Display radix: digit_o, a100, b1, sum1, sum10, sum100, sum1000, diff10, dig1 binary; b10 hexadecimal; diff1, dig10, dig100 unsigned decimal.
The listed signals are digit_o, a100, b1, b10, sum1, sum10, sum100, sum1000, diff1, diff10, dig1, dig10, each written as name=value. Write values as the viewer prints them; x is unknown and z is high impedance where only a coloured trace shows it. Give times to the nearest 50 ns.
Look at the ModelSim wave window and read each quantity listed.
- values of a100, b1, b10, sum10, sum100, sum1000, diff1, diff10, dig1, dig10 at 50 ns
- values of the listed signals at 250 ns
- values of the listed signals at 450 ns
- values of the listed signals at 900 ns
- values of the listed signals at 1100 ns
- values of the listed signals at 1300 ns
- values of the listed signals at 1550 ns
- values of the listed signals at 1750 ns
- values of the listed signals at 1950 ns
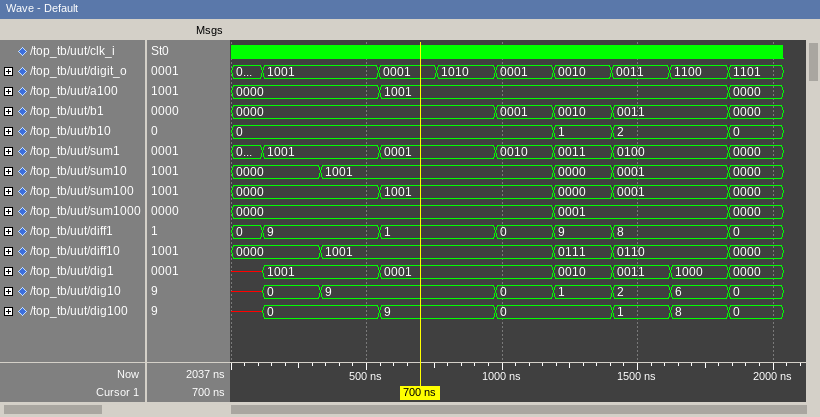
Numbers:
a100=0000, b1=0000, b10=0, sum10=0000, sum100=0000, sum1000=0000, diff1=0, diff10=0000, dig1=x, dig10=x
digit_o=1001, a100=0000, b1=0000, b10=0, sum1=1001, sum10=0000, sum100=0000, sum1000=0000, diff1=9, diff10=0000, dig1=1001, dig10=0
digit_o=1001, a100=0000, b1=0000, b10=0, sum1=1001, sum10=1001, sum100=0000, sum1000=0000, diff1=9, diff10=1001, dig1=1001, dig10=9
digit_o=1010, a100=1001, b1=0000, b10=0, sum1=0001, sum10=1001, sum100=1001, sum1000=0000, diff1=1, diff10=1001, dig1=0001, dig10=9
digit_o=0001, a100=1001, b1=0001, b10=0, sum1=0010, sum10=1001, sum100=1001, sum1000=0000, diff1=0, diff10=1001, dig1=0001, dig10=0
digit_o=0010, a100=1001, b1=0010, b10=1, sum1=0011, sum10=0000, sum100=0000, sum1000=0001, diff1=9, diff10=0111, dig1=0010, dig10=1
digit_o=0011, a100=1001, b1=0011, b10=2, sum1=0100, sum10=0001, sum100=0001, sum1000=0001, diff1=8, diff10=0110, dig1=0011, dig10=2
digit_o=1100, a100=1001, b1=0011, b10=2, sum1=0100, sum10=0001, sum100=0001, sum1000=0001, diff1=8, diff10=0110, dig1=1000, dig10=6
digit_o=1101, a100=0000, b1=0000, b10=0, sum1=0000, sum10=0000, sum100=0000, sum1000=0000, diff1=0, diff10=0000, dig1=0000, dig10=0
